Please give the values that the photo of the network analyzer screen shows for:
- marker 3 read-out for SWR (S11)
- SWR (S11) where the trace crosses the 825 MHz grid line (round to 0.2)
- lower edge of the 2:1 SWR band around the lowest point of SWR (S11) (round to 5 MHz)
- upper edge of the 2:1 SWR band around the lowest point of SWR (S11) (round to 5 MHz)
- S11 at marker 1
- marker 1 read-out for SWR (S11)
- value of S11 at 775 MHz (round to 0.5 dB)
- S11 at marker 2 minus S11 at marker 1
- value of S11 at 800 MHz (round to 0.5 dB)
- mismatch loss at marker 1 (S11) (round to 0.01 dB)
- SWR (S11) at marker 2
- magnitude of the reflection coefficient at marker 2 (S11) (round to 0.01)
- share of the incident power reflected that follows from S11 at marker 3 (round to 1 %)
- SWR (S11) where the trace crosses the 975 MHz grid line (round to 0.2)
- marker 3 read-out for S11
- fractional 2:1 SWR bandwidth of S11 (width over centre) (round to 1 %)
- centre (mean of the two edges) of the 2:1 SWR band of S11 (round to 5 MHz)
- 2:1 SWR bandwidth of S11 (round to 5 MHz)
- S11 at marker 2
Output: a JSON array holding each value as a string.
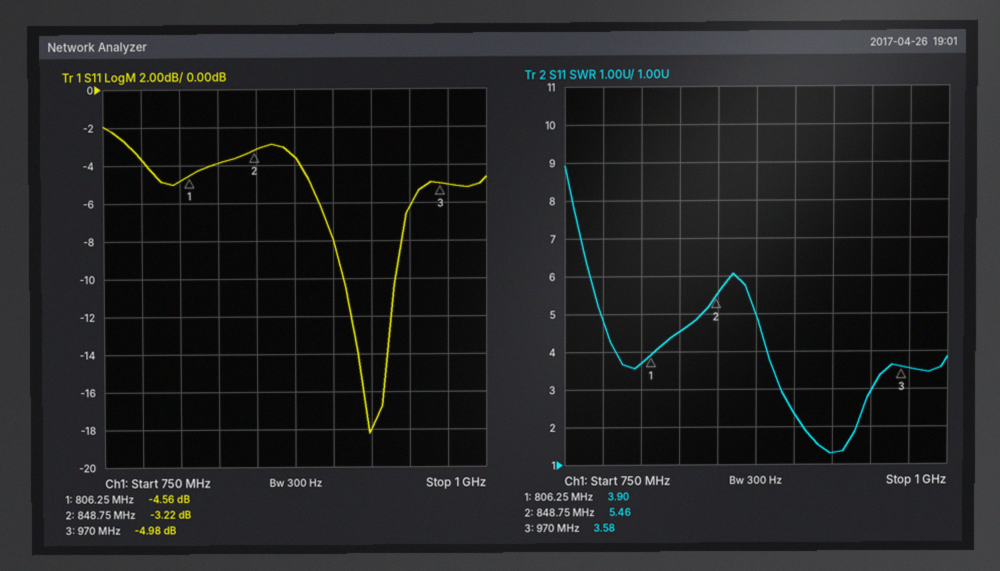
["3.58", "4.6", "905 MHz", "940 MHz", "-4.56 dB", "3.90", "-3.5 dB", "1.34 dB", "-5.0 dB", "1.87 dB", "5.46", "0.69", "32 %", "3.6", "-4.98 dB", "4 %", "925 MHz", "35 MHz", "-3.22 dB"]
